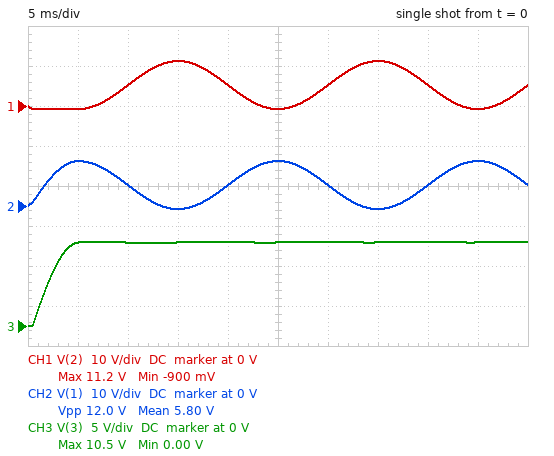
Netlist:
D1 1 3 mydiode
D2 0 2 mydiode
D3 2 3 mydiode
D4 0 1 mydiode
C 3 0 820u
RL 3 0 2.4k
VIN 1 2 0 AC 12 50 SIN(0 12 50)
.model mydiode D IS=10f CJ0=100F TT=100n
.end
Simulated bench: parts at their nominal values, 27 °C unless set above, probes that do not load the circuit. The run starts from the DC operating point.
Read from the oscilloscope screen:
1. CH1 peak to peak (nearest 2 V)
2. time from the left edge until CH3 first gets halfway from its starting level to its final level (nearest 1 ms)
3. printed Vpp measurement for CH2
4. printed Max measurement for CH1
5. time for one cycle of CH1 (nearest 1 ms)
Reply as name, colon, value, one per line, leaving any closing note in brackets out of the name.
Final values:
CH1 peak to peak: 12 V
time from the left edge until CH3 first gets halfway from its starting level to its final level: 2 ms
printed Vpp measurement for CH2: 12.0 V
printed Max measurement for CH1: 11.2 V
time for one cycle of CH1: 20 ms
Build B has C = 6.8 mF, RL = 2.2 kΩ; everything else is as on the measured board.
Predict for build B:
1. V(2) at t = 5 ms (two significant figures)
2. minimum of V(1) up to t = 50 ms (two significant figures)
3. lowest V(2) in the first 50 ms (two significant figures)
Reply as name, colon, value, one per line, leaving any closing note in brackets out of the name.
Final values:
V(2) at t = 5 ms: -840 mV
minimum of V(1) up to t = 50 ms: -820 mV
lowest V(2) in the first 50 ms: -920 mV
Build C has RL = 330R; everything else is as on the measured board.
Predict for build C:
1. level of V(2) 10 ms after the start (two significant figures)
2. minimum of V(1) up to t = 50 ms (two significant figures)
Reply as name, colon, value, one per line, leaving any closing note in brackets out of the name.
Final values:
level of V(2) 10 ms after the start: 5.1 V
minimum of V(1) up to t = 50 ms: -820 mV
